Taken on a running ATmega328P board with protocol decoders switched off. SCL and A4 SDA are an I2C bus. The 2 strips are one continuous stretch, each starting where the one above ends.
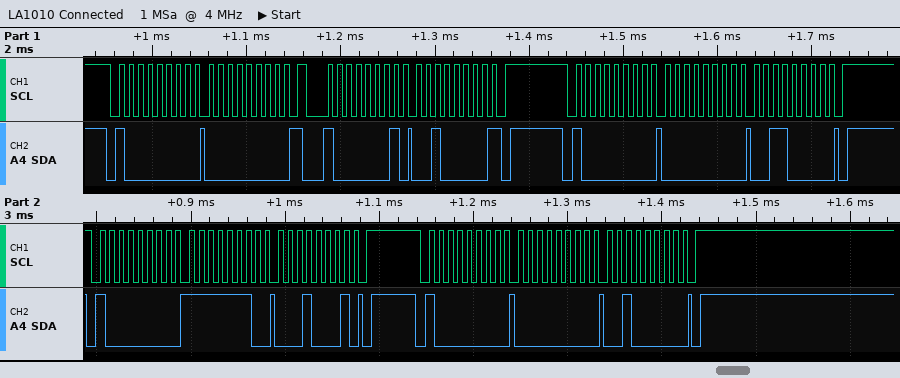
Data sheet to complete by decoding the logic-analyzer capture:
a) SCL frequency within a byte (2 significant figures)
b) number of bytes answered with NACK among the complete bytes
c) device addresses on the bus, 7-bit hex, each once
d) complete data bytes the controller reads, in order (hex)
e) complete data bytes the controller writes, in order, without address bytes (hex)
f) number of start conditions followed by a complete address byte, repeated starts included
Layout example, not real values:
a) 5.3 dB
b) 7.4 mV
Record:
a) 100 kHz
b) 1
c) 0x40
d) 20
e) 00 00 30 FE 11 00 20
f) 5
